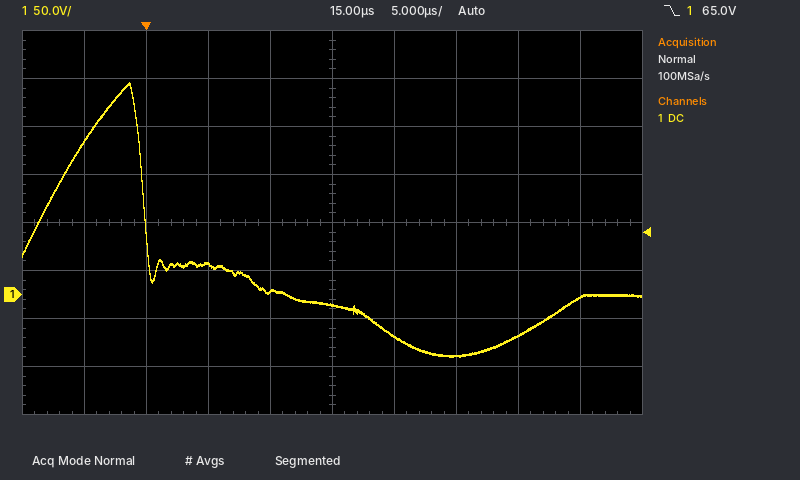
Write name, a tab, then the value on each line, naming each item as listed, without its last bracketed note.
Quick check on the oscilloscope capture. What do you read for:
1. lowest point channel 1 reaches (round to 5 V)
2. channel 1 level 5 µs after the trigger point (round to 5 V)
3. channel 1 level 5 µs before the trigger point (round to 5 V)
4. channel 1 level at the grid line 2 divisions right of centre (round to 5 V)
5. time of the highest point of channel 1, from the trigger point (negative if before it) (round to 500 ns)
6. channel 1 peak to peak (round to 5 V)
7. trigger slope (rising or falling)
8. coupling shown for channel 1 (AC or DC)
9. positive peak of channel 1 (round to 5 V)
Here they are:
lowest point channel 1 reaches	-65 V
channel 1 level 5 µs after the trigger point	30 V
channel 1 level 5 µs before the trigger point	160 V
channel 1 level at the grid line 2 divisions right of centre	-65 V
time of the highest point of channel 1, from the trigger point (negative if before it)	-1.5 µs
channel 1 peak to peak	285 V
trigger slope	falling
coupling shown for channel 1	DC
positive peak of channel 1	220 V
